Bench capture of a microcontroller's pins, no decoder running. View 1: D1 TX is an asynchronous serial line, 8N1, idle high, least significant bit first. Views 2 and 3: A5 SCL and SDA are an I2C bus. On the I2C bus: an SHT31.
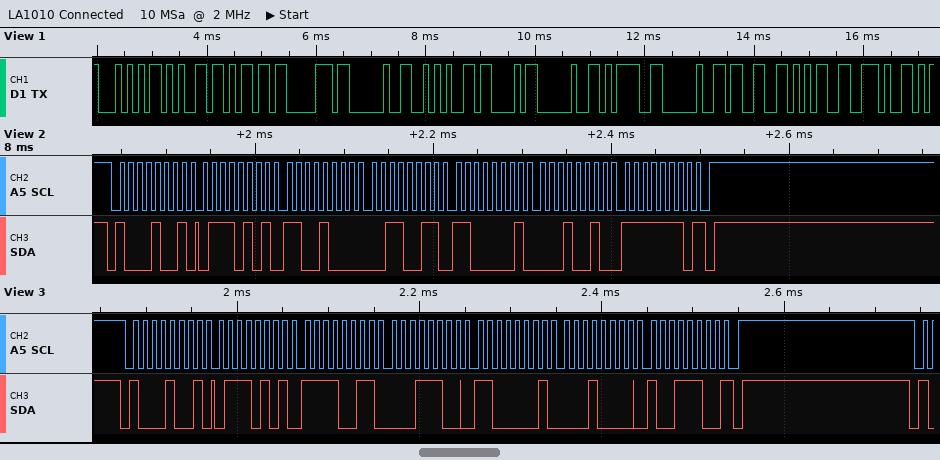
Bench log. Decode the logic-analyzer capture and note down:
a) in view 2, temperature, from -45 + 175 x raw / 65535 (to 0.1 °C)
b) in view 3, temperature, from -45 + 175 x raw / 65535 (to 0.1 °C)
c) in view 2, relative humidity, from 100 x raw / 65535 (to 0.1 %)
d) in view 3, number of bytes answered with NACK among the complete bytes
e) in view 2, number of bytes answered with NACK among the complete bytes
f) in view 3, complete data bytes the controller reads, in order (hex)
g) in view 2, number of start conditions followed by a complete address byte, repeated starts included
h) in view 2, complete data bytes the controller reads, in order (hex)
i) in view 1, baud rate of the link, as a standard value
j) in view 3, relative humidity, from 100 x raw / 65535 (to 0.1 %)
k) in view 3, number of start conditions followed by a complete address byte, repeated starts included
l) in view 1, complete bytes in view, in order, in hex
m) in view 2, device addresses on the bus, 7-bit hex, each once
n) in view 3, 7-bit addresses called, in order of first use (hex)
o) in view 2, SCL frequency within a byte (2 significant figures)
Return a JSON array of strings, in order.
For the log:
["35.5 °C", "35.6 °C", "75.4 %", "1", "1", "75 F3 1C C1 10 9C", "1", "75 C8 33 C1 12 FE", "9600 baud", "75.4 %", "1", "54 65 6D 70 20 2A 43 20 3D 20 33 35 2E", "0x44", "0x44", "100 kHz"]
